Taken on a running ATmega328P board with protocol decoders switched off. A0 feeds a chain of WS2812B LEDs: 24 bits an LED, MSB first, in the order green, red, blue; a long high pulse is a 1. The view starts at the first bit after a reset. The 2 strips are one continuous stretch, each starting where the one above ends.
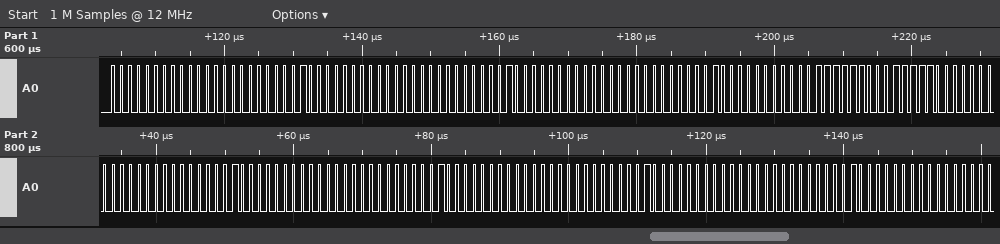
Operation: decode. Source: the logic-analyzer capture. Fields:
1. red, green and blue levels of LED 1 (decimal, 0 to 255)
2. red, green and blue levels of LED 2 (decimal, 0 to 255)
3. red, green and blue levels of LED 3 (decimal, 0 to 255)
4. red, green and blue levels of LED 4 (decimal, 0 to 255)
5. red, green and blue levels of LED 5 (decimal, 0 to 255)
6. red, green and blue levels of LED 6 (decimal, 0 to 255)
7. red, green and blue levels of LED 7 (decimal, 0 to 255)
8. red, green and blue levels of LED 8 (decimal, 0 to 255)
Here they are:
0, 0, 2
0, 0, 2
0, 0, 2
63, 0, 31
0, 0, 2
0, 0, 2
0, 0, 2
0, 0, 2
